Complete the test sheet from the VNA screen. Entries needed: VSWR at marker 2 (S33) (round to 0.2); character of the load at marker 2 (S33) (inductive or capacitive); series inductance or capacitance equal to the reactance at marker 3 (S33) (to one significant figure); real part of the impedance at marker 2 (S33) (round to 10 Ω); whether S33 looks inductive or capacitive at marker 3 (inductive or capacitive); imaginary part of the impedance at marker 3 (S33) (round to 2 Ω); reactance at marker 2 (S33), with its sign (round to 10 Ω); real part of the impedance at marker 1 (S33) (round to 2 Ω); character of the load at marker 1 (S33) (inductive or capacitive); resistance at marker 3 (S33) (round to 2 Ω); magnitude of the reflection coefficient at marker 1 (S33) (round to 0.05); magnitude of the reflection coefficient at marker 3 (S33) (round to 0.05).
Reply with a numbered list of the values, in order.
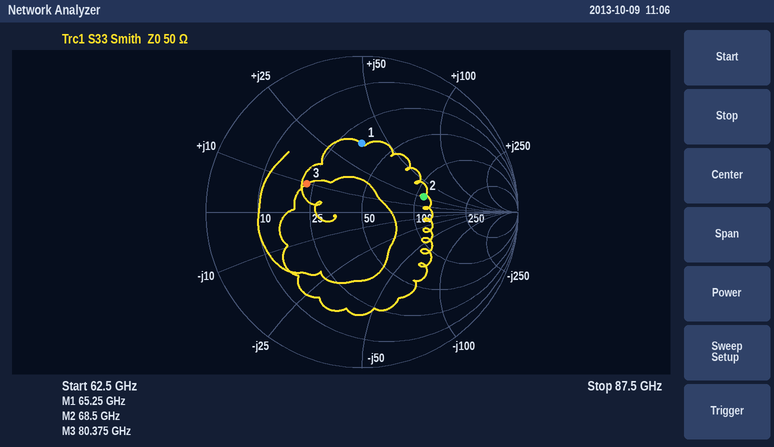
1. 2.4
2. inductive
3. 20 pH
4. 110 Ω
5. inductive
6. +10 Ω
7. +30 Ω
8. 34 Ω
9. inductive
10. 22 Ω
11. 0.45
12. 0.40
